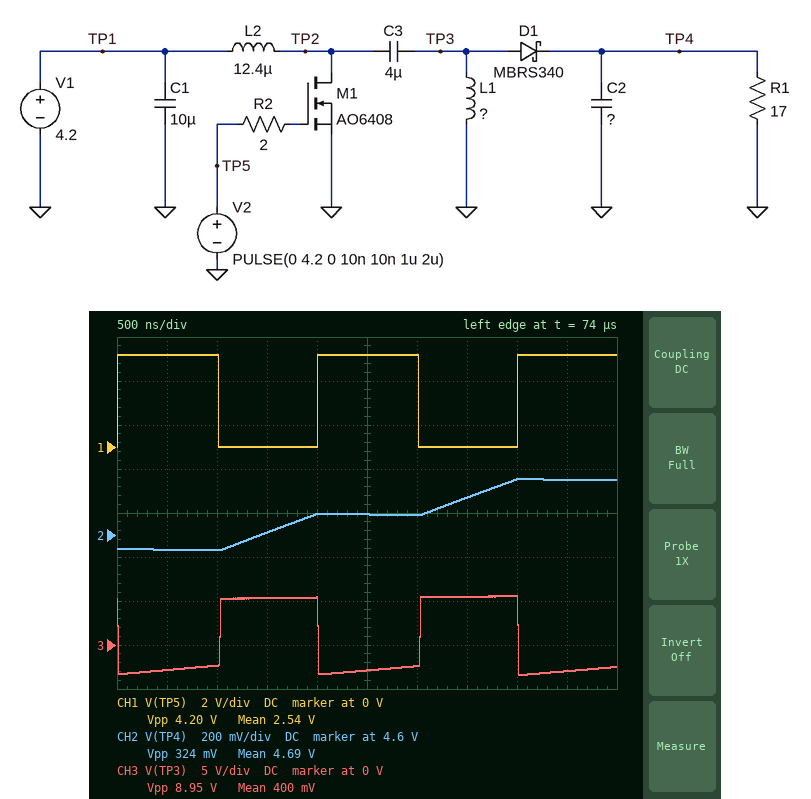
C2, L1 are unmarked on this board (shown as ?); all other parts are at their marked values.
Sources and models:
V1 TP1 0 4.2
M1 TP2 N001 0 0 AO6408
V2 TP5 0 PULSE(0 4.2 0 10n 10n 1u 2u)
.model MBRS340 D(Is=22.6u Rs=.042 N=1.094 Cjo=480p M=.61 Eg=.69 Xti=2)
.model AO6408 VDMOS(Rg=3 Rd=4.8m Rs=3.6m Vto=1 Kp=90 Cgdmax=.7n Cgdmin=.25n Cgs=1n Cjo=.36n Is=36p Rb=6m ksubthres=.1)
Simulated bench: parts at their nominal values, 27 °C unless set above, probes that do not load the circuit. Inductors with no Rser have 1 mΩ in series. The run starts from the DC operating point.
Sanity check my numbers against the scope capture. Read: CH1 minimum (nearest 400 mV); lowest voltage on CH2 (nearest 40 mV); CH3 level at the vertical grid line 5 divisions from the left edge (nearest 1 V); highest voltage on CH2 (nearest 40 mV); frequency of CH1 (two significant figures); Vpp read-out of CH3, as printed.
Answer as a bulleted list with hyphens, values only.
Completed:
- 0 V
- 4.52 V
- -3 V
- 4.84 V
- 500 kHz
- 8.95 V
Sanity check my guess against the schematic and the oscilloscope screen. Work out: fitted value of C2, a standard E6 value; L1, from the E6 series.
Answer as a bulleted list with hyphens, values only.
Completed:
- 47 µF
- 22 µH
